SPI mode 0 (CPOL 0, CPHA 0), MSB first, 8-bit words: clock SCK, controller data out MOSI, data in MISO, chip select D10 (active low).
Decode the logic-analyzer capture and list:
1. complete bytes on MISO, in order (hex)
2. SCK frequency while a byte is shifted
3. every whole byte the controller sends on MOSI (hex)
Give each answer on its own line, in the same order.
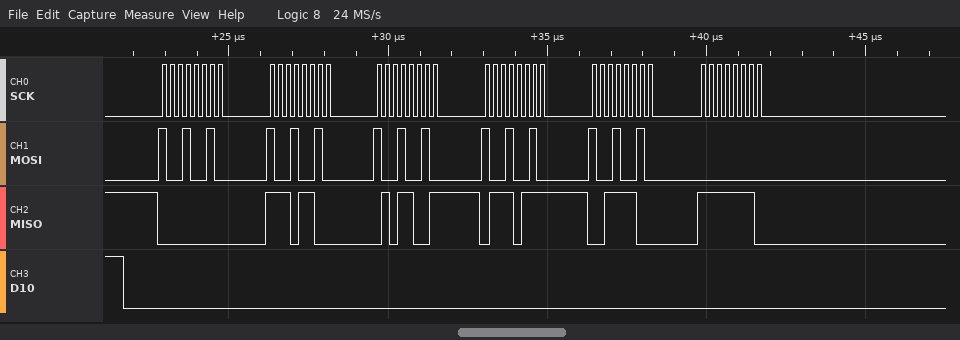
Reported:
0x00 0xEC 0x59 0x77 0x3C 0xFE
4 MHz
0x92 0x92 0x92 0x92 0x92 0x00
